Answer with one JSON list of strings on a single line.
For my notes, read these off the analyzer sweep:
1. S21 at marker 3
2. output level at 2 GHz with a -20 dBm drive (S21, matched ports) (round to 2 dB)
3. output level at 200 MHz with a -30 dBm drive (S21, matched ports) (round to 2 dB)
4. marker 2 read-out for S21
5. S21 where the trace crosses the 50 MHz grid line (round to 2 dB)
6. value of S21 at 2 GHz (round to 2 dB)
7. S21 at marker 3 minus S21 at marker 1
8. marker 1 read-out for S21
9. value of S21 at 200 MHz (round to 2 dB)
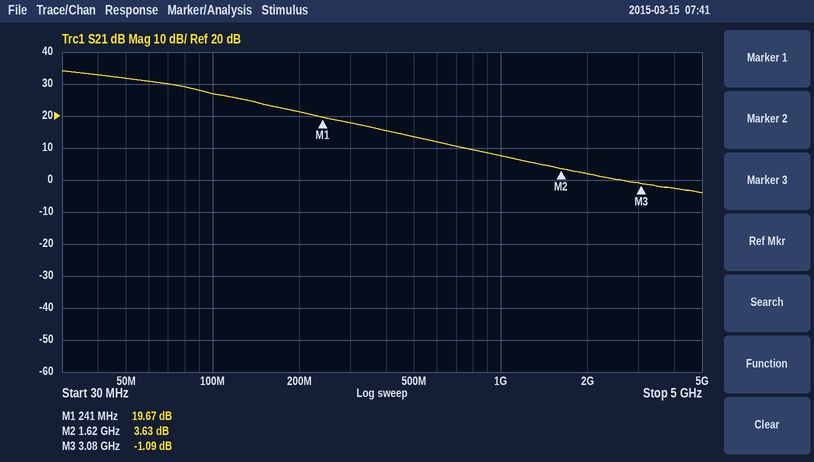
["-1.09 dB", "-18 dBm", "-8 dBm", "3.63 dB", "32 dB", "2 dB", "-20.76 dB", "19.67 dB", "22 dB"]
